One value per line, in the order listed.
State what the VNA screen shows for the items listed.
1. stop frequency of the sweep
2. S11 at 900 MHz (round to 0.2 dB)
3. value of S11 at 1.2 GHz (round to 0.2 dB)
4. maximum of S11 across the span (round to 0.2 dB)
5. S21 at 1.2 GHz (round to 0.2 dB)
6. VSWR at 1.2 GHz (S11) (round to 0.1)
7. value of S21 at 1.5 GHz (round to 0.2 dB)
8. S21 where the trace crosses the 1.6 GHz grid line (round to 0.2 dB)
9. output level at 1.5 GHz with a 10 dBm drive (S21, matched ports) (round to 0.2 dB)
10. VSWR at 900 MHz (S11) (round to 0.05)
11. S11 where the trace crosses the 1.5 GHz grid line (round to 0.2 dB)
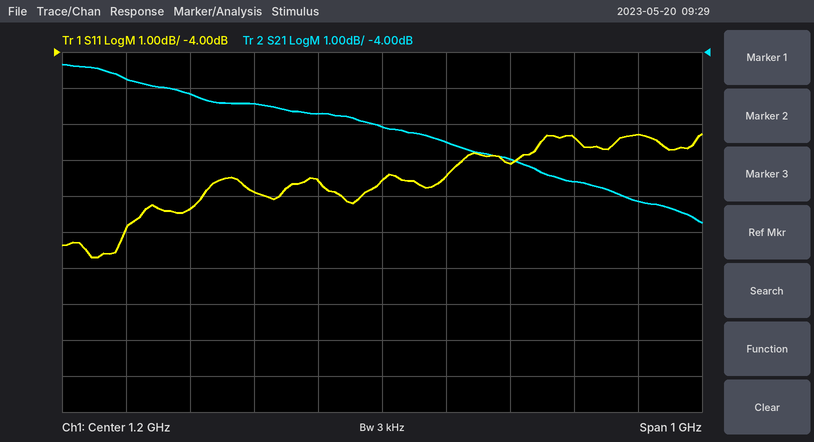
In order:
1.7 GHz
-8.4 dB
-7.6 dB
-6.2 dB
-6.0 dB
2.4
-7.6 dB
-8.2 dB
2.4 dBm
2.25
-6.4 dB
